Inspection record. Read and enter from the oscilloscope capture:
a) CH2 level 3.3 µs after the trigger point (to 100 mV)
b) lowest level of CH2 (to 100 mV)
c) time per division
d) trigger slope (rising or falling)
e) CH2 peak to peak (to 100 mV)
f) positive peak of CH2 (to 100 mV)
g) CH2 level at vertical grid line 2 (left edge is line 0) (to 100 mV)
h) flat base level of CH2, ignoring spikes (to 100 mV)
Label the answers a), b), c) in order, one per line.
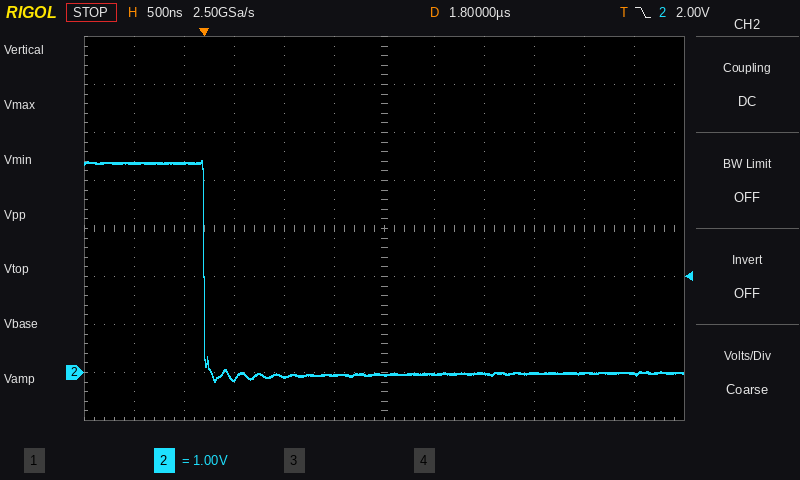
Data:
a) 0.0 V
b) -200 mV
c) 500 ns
d) falling
e) 4.6 V
f) 4.4 V
g) 4.4 V
h) 0.0 V
